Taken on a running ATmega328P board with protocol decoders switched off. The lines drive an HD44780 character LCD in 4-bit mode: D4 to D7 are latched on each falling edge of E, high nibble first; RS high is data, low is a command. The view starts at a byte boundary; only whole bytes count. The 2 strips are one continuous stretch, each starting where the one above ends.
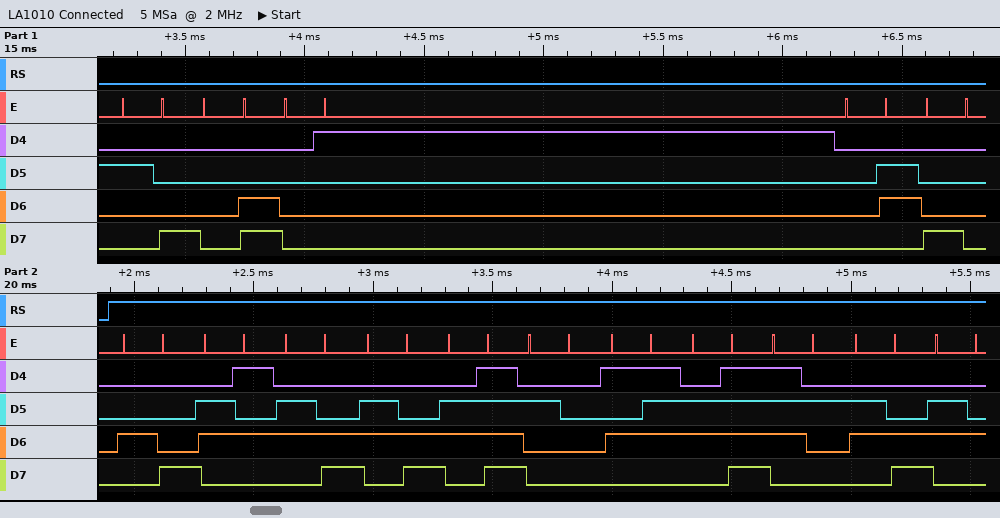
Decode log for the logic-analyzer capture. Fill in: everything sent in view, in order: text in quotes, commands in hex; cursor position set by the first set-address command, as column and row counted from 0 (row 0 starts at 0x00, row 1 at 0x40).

0x28 0x0C 0x01 0x06 0x80 "Hello World"
column 0, row 0
